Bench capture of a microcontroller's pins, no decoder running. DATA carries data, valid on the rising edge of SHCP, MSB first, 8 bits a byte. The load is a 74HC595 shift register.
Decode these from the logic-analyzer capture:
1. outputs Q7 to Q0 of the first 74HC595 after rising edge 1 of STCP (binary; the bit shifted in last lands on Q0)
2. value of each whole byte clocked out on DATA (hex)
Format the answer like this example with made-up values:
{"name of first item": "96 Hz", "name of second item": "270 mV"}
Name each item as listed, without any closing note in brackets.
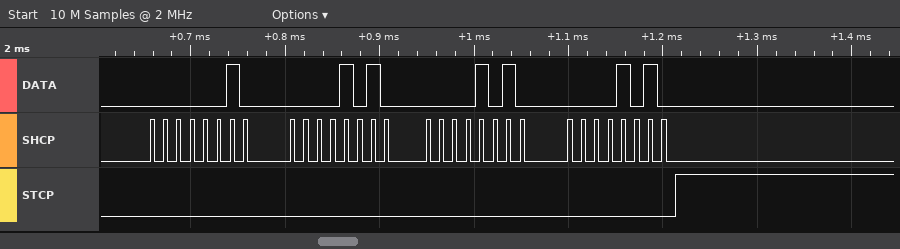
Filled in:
{"outputs Q7 to Q0 of the first 74HC595 after rising edge 1 of STCP": "00001010", "value of each whole byte clocked out on DATA": "02 0A 0A 0A"}
